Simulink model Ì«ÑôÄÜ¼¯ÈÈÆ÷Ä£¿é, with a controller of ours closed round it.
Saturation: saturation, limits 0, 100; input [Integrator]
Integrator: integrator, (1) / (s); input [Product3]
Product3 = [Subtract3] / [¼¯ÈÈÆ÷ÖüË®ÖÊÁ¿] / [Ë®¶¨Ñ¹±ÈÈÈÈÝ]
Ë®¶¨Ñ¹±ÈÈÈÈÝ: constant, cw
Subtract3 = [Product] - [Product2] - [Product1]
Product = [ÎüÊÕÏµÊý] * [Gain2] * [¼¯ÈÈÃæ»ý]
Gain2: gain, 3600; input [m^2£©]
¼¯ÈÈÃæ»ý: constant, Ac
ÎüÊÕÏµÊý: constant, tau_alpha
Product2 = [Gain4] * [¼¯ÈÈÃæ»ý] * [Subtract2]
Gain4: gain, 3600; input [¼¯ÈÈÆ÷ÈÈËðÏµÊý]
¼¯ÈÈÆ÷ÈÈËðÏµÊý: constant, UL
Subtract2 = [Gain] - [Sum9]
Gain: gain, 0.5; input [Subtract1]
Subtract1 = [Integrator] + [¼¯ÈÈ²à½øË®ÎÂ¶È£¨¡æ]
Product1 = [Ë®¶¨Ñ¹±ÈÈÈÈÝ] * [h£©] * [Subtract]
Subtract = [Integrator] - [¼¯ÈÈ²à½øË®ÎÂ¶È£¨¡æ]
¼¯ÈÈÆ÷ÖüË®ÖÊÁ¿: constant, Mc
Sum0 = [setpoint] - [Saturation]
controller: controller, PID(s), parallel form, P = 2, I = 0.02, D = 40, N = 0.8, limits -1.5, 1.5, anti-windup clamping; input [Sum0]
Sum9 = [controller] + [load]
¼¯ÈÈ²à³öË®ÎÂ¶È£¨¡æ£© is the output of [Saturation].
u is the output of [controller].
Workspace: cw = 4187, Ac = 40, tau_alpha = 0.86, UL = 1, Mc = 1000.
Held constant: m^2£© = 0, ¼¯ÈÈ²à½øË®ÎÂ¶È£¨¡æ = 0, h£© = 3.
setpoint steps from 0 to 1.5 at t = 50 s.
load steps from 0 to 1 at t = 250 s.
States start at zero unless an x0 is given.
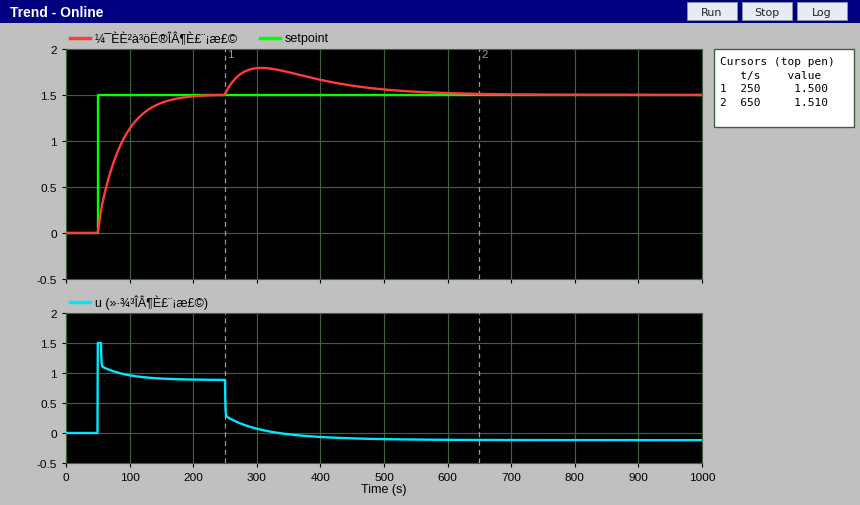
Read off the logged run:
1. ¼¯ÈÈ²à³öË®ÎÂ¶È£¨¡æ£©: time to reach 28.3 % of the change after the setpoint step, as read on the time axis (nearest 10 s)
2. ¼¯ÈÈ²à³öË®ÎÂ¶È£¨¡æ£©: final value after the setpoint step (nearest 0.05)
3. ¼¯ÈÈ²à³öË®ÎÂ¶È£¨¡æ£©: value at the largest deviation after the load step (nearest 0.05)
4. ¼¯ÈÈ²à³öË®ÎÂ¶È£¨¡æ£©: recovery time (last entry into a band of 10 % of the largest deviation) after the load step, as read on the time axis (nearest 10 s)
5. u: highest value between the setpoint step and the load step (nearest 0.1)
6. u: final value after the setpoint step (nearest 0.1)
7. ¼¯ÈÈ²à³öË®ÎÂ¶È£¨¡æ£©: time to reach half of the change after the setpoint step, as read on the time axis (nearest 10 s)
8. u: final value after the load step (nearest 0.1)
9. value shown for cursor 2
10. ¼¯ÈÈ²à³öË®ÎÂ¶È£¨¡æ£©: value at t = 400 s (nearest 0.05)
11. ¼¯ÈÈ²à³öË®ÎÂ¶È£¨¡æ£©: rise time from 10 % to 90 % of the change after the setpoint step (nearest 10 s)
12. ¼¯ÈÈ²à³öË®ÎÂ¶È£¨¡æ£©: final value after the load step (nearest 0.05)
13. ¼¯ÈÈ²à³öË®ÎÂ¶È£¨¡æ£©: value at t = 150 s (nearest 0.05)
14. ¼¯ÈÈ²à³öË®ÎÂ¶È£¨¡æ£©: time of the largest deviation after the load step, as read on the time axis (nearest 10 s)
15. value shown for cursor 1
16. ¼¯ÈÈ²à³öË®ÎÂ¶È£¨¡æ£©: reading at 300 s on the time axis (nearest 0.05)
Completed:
60 s
1.50
1.80
570 s
1.5
0.9
70 s
-0.1
1.510
1.65
80 s
1.50
1.40
310 s
1.500
1.80
